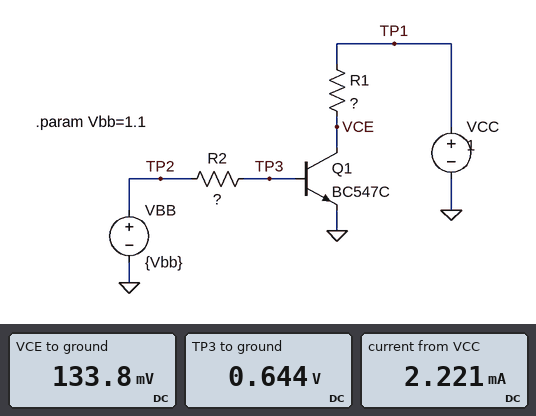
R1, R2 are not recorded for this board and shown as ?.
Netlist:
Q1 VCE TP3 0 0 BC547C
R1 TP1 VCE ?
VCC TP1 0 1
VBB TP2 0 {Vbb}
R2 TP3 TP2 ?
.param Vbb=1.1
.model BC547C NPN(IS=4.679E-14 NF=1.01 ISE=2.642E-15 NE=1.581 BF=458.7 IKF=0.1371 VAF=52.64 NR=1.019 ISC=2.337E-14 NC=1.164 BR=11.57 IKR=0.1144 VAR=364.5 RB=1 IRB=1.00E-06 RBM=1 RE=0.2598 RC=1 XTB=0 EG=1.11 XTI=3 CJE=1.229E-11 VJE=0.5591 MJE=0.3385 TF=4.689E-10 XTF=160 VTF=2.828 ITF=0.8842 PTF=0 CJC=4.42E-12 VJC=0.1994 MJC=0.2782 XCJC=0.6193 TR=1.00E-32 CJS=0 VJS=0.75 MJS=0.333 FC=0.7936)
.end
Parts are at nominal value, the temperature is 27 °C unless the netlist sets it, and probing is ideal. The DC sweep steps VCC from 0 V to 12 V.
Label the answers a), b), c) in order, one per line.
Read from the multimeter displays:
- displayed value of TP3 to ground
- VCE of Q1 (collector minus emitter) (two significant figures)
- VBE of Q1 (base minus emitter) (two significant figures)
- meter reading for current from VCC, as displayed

a) 0.644 V
b) 130 mV
c) 640 mV
d) 2.221 mA
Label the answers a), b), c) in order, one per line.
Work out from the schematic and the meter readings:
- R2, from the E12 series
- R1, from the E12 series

a) 68 kΩ
b) 390 Ω
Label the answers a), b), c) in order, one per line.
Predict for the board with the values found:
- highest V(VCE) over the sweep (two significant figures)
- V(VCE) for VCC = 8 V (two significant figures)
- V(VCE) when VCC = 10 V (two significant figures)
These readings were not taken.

a) 11 V
b) 6.7 V
c) 8.7 V
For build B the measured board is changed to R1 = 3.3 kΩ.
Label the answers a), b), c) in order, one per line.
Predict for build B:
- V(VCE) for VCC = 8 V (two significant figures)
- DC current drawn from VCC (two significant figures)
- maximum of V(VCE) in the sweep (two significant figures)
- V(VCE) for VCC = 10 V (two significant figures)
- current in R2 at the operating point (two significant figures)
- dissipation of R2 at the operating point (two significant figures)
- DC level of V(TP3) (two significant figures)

a) 140 mV
b) 290 µA
c) 2.0 V
d) 330 mV
e) 7.4 µA
f) 3.8 µW
g) 590 mV
